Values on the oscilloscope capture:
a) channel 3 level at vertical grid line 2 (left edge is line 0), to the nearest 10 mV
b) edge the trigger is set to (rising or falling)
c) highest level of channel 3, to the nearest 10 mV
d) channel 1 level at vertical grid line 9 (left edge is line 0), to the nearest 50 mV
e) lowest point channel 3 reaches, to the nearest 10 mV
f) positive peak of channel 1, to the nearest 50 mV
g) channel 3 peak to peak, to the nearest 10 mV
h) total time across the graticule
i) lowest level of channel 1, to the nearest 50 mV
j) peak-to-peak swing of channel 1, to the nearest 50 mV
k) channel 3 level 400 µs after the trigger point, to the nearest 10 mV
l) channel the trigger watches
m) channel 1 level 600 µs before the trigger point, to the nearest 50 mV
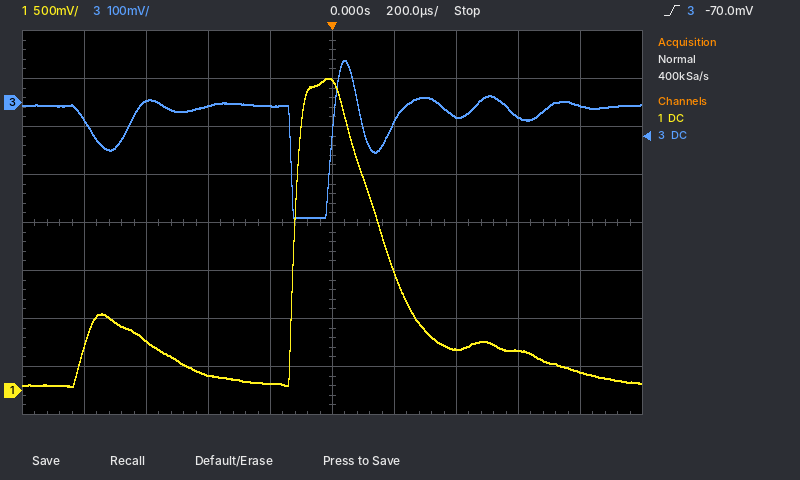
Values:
0 mV
rising
90 mV
200 mV
-240 mV
3.25 V
330 mV
2 ms
50 mV
3.20 V
-30 mV
channel 3
500 mV
